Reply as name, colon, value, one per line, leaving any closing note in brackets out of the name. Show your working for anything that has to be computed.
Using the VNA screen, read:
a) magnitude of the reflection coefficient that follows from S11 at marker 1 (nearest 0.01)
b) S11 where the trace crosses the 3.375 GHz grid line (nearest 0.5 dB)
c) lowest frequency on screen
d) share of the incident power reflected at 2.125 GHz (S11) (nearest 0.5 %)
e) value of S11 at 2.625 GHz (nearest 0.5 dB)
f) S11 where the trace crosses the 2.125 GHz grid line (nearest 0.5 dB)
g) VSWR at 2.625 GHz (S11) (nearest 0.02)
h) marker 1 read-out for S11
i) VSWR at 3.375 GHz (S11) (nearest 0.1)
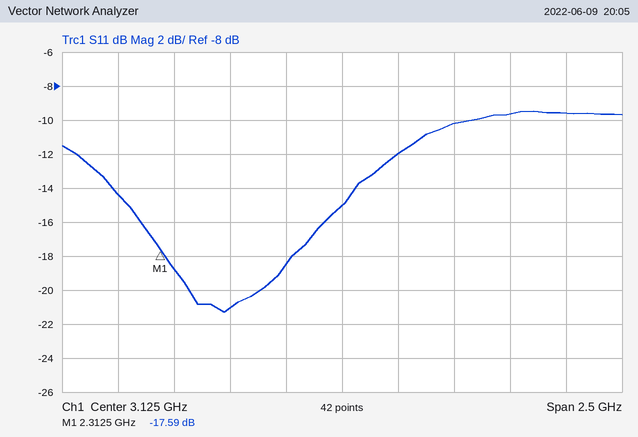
magnitude of the reflection coefficient that follows from S11 at marker 1: 10^(-17.59/20) ≈ 0.13
S11 where the trace crosses the 3.375 GHz grid line: -12.0 dB
lowest frequency on screen: 1.875 GHz
share of the incident power reflected at 2.125 GHz (S11): 10^(-14.5/10) ≈ 3.5 %
value of S11 at 2.625 GHz: -21.0 dB
S11 where the trace crosses the 2.125 GHz grid line: -14.5 dB
VSWR at 2.625 GHz (S11): |Γ| = 10^(-21/20) = 0.0891; VSWR = (1 + 0.0891)/(1 − 0.0891) ≈ 1.20
marker 1 read-out for S11: -17.59 dB
VSWR at 3.375 GHz (S11): |Γ| = 10^(-12/20) = 0.2512; VSWR = (1 + 0.2512)/(1 − 0.2512) ≈ 1.7
